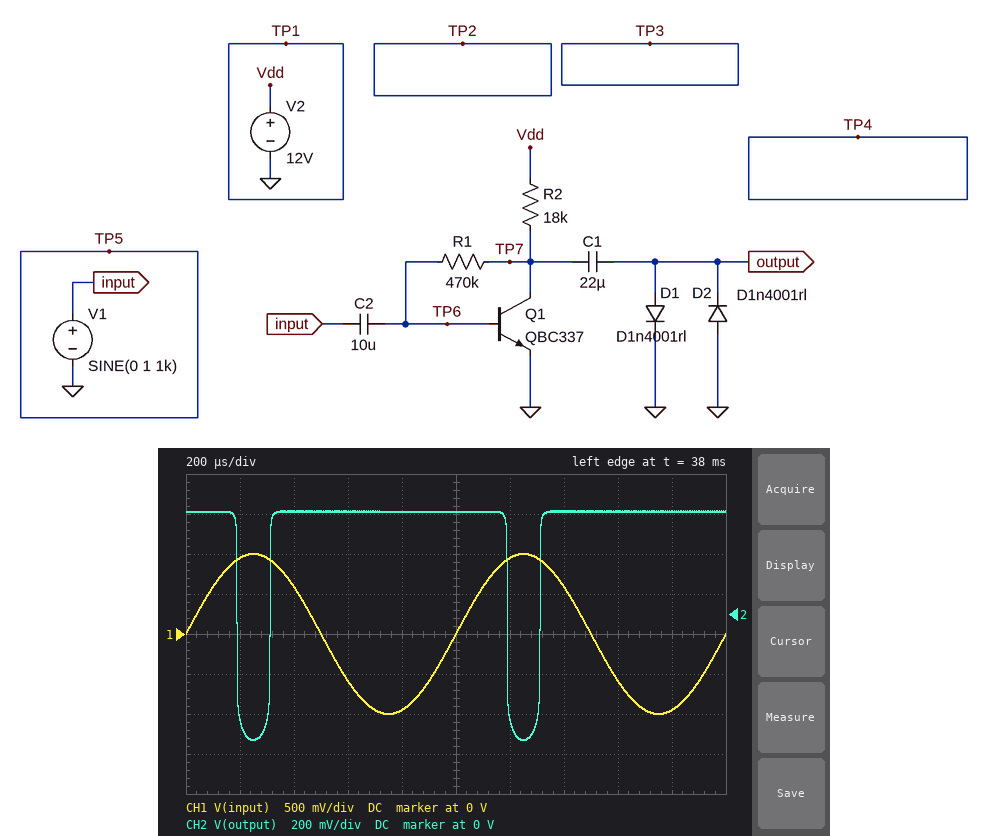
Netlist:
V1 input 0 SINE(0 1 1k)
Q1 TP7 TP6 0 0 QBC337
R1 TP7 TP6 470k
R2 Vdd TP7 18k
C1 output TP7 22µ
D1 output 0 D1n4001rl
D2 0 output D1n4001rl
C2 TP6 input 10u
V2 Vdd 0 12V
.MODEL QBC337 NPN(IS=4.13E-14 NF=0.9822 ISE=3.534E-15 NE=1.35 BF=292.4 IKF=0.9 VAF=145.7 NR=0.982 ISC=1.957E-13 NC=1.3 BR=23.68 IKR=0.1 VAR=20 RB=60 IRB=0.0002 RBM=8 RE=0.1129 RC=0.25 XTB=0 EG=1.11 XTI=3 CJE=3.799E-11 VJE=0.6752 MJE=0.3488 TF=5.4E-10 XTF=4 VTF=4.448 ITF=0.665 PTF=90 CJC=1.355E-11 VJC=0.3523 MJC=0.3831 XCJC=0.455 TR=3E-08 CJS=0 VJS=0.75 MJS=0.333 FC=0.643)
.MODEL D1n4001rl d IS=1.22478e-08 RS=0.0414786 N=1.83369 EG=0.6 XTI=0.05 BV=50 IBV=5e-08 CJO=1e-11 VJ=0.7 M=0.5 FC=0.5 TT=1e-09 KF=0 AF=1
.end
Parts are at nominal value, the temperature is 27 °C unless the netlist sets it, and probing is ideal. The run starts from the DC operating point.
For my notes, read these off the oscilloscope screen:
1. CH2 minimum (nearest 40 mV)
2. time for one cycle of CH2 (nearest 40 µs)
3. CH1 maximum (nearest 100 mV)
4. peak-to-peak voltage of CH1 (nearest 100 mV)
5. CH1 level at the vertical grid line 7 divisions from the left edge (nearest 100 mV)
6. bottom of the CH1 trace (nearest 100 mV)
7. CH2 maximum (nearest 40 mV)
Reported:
-640 mV
1.00 ms
1.0 V
2.0 V
600 mV
-1.0 V
520 mV
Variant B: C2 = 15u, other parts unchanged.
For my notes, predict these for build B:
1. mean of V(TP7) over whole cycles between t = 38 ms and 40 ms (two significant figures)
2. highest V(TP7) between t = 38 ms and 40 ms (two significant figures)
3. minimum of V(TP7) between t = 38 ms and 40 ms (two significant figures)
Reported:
1.0 V
1.2 V
39 mV
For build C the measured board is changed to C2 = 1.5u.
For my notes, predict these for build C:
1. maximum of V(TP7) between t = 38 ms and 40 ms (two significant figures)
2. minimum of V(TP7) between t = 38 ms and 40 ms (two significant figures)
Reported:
1.3 V
92 mV
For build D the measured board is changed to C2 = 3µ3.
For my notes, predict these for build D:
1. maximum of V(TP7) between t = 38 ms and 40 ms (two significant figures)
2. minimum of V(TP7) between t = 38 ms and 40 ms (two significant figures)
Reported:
1.3 V
110 mV
